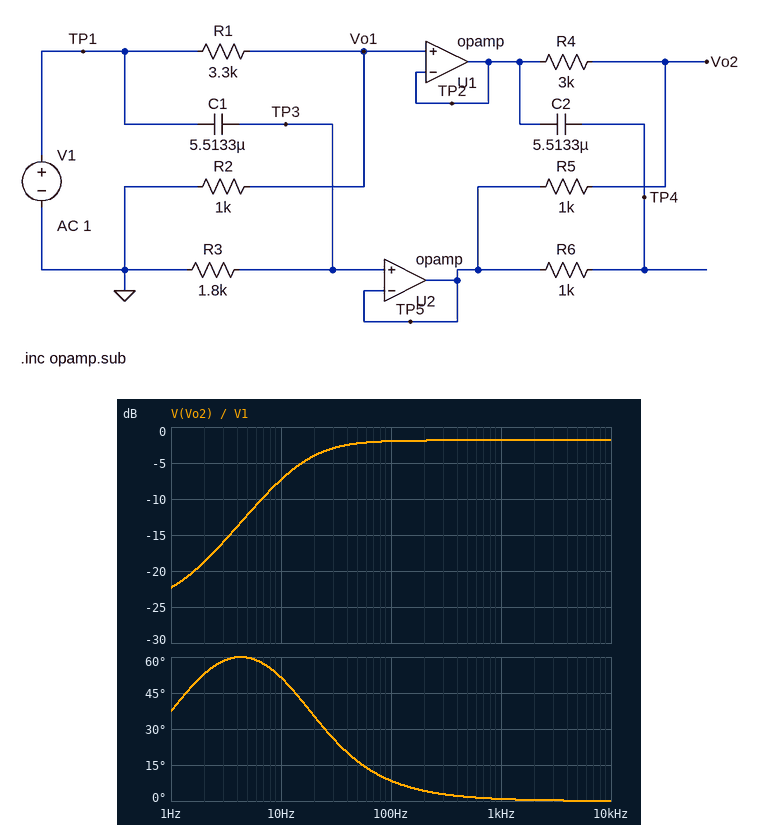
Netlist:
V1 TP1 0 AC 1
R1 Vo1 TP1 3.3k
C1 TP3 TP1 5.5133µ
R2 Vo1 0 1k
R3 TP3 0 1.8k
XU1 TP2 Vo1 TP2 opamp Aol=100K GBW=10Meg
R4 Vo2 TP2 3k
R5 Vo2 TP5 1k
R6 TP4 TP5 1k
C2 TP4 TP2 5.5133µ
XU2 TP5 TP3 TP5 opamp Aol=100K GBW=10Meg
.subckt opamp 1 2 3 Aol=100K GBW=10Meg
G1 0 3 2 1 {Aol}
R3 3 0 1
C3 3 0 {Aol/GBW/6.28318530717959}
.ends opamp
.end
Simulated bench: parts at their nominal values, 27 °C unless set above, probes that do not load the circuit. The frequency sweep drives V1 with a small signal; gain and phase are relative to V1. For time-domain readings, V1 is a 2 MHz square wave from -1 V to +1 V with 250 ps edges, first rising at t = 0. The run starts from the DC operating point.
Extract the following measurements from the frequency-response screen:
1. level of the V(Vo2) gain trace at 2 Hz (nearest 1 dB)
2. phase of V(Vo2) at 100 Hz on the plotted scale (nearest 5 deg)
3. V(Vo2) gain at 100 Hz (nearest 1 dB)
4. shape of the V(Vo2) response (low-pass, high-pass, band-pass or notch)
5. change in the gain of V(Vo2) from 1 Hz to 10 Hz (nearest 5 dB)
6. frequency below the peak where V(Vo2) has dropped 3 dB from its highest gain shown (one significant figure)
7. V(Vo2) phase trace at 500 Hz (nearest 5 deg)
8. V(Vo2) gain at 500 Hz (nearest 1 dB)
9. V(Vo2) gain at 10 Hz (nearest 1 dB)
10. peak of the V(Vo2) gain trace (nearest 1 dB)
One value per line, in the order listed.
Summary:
-19 dB
10 deg
-2 dB
high-pass
15 dB
20 Hz
0 deg
-2 dB
-7 dB
-2 dB
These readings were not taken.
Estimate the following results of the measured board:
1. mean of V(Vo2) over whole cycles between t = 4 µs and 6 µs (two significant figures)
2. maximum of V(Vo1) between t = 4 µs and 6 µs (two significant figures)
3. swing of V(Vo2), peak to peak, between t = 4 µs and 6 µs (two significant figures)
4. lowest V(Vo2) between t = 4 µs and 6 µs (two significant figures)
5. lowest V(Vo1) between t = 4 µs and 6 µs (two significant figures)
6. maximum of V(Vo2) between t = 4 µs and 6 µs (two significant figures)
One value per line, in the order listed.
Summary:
750 mV
230 mV
1.6 V
-59 mV
-230 mV
1.6 V
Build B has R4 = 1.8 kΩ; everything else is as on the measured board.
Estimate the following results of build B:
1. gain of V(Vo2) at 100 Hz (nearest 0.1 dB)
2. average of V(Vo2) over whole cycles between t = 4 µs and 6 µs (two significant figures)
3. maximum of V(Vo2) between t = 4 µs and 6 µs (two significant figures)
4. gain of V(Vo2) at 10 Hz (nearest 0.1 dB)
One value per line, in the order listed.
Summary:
-2.9 dB
640 mV
1.4 V
-8.2 dB
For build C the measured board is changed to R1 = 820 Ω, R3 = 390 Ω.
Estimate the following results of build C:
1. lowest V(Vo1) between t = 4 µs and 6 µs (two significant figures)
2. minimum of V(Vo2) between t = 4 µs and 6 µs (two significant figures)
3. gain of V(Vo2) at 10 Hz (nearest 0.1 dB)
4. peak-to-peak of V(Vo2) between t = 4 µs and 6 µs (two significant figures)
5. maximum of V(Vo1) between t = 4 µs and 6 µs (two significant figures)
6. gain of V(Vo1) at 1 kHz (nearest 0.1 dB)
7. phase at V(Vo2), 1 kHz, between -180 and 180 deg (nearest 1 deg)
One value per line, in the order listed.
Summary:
-550 mV
-140 mV
-14.9 dB
1.8 V
550 mV
-5.2 dB
4 deg
